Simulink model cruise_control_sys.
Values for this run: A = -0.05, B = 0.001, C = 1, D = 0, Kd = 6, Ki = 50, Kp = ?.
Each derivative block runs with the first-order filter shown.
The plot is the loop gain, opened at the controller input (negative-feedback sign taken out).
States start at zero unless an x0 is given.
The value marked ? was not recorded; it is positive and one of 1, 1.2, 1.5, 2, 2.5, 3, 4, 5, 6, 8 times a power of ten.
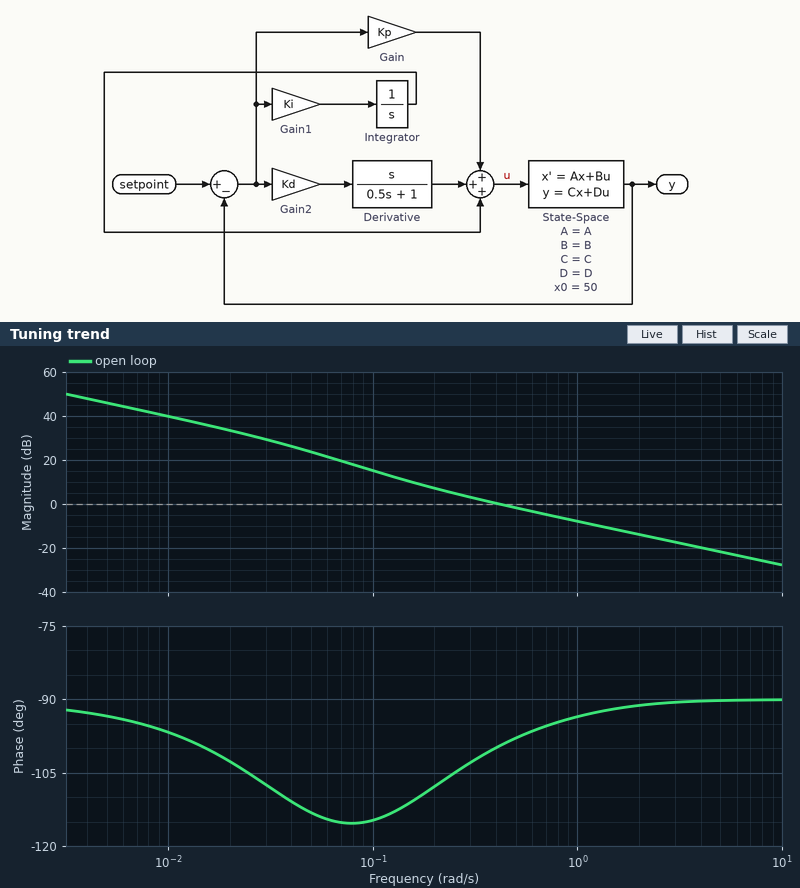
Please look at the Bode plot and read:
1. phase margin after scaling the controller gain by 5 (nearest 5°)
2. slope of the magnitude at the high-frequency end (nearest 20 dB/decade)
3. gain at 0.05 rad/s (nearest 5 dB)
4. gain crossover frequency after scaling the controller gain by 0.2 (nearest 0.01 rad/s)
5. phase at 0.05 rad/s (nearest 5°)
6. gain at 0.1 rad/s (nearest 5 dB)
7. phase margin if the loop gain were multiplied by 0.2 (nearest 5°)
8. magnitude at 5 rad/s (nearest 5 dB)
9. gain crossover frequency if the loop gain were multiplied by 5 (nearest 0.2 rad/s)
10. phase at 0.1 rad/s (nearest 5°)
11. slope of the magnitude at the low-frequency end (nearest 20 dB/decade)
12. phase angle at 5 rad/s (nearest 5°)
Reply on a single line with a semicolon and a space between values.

90°; -20 dB/decade; 25 dB; 0.11 rad/s; -115°; 15 dB; 65°; -20 dB; 2.0 rad/s; -115°; -20 dB/decade; -90°
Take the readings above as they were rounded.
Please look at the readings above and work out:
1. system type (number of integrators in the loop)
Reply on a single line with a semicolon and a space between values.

1
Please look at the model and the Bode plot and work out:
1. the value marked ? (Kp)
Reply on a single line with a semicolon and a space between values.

400
